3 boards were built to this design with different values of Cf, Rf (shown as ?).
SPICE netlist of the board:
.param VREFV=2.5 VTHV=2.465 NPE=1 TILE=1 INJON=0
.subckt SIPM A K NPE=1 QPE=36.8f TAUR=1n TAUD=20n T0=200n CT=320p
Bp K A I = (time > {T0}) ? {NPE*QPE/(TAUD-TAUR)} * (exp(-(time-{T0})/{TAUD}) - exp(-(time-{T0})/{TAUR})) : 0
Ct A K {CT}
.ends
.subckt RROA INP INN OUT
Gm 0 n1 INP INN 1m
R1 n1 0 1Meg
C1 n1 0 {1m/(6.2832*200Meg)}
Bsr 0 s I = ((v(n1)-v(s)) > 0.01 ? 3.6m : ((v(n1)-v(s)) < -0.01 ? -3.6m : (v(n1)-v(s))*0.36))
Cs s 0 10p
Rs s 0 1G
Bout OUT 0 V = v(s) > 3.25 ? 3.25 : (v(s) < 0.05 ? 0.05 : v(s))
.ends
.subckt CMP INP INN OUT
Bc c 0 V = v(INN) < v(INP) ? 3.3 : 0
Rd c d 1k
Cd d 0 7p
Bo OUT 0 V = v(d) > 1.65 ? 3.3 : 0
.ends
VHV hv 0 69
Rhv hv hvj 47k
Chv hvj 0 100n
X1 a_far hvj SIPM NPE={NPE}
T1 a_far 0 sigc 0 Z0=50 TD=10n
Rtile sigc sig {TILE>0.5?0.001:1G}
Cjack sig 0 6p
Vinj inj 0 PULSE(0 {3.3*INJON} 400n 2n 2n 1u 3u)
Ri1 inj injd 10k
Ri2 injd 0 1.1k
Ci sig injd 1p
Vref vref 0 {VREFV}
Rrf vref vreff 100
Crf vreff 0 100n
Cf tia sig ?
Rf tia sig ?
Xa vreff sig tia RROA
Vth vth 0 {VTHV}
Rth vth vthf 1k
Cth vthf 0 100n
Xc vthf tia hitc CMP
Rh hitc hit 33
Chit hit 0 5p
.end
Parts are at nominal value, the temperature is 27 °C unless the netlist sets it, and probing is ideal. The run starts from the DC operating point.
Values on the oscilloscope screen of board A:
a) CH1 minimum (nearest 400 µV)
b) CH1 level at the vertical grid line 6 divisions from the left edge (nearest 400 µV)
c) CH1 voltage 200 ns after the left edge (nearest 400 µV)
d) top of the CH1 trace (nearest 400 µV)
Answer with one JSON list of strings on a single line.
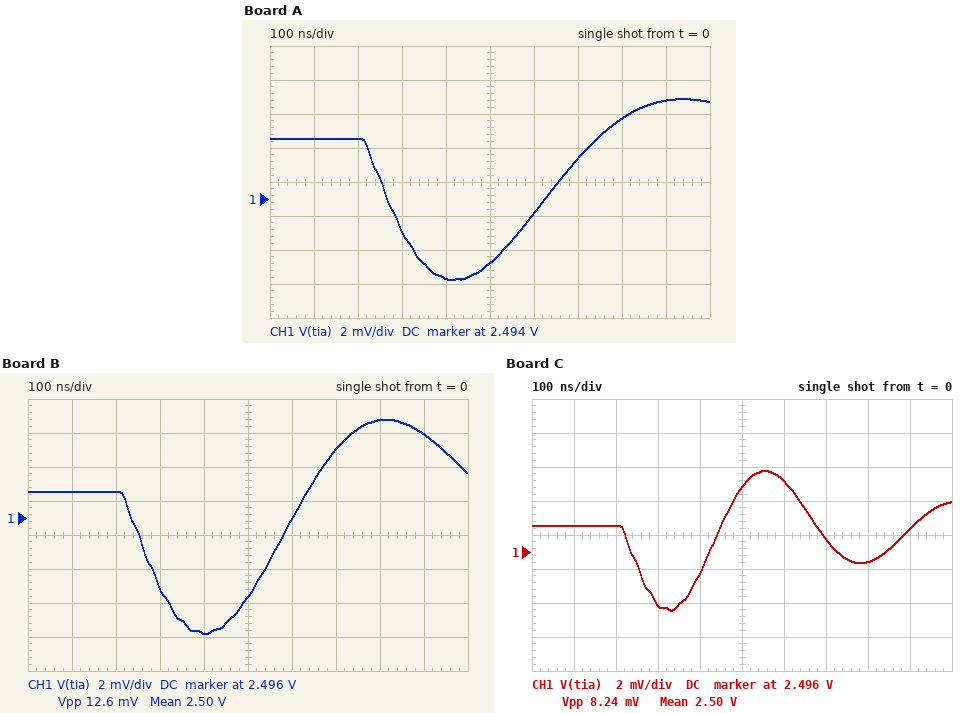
["2.4892 V", "2.4932 V", "2.4976 V", "2.5000 V"]
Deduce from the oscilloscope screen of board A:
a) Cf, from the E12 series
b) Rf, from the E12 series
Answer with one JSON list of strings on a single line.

["1.5 pF", "56 kΩ"]
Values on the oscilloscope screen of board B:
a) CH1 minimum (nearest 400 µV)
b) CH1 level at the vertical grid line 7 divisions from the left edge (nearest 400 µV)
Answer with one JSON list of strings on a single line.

["2.4892 V", "2.5000 V"]
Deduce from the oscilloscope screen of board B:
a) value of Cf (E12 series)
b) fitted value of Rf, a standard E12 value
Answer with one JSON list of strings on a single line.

["820 fF", "39 kΩ"]
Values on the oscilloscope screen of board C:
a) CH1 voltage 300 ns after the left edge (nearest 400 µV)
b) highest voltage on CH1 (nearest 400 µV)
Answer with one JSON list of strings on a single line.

["2.4928 V", "2.5008 V"]
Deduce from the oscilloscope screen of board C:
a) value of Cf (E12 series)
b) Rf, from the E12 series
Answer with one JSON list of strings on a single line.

["1 pF", "12 kΩ"]
